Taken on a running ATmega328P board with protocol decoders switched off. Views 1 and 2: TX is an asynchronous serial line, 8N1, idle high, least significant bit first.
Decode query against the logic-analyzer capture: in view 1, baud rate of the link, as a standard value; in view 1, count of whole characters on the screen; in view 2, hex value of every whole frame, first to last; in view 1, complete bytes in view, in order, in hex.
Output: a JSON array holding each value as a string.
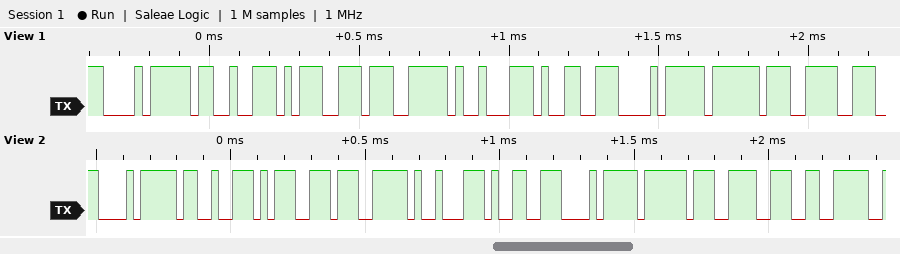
["38400 baud", "9", "0xE8 0x93 0x9D 0xE7 0x89 0x99 0xE8 0xBF 0x9E 0xE6", "0xE8 0x93 0x9D 0xE7 0x89 0x99 0xE8 0xBF 0x9E"]
